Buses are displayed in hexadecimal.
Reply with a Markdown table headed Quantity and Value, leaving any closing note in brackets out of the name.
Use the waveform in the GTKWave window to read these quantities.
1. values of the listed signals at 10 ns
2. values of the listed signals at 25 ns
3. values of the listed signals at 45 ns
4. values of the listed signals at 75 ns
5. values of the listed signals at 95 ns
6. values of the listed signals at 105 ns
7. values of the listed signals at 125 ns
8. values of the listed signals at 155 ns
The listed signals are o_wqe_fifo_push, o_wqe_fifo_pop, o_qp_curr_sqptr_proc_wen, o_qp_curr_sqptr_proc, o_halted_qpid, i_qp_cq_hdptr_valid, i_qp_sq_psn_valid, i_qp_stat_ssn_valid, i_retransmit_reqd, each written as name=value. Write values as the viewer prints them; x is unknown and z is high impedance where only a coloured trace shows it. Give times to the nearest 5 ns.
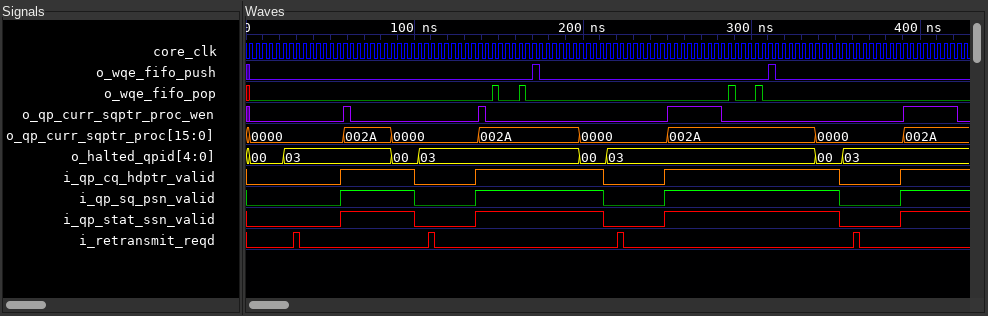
| Quantity | Value |
|---|---|
| values of the listed signals at 10 ns | o_wqe_fifo_push=0, o_wqe_fifo_pop=0, o_qp_curr_sqptr_proc_wen=0, o_qp_curr_sqptr_proc=0000, o_halted_qpid=00, i_qp_cq_hdptr_valid=0, i_qp_sq_psn_valid=0, i_qp_stat_ssn_valid=0, i_retransmit_reqd=0 |
| values of the listed signals at 25 ns | o_wqe_fifo_push=0, o_wqe_fifo_pop=0, o_qp_curr_sqptr_proc_wen=0, o_qp_curr_sqptr_proc=0000, o_halted_qpid=03, i_qp_cq_hdptr_valid=0, i_qp_sq_psn_valid=0, i_qp_stat_ssn_valid=0, i_retransmit_reqd=0 |
| values of the listed signals at 45 ns | o_wqe_fifo_push=0, o_wqe_fifo_pop=0, o_qp_curr_sqptr_proc_wen=0, o_qp_curr_sqptr_proc=0000, o_halted_qpid=03, i_qp_cq_hdptr_valid=0, i_qp_sq_psn_valid=0, i_qp_stat_ssn_valid=0, i_retransmit_reqd=0 |
| values of the listed signals at 75 ns | o_wqe_fifo_push=0, o_wqe_fifo_pop=0, o_qp_curr_sqptr_proc_wen=0, o_qp_curr_sqptr_proc=002A, o_halted_qpid=03, i_qp_cq_hdptr_valid=1, i_qp_sq_psn_valid=1, i_qp_stat_ssn_valid=1, i_retransmit_reqd=0 |
| values of the listed signals at 95 ns | o_wqe_fifo_push=0, o_wqe_fifo_pop=0, o_qp_curr_sqptr_proc_wen=0, o_qp_curr_sqptr_proc=0000, o_halted_qpid=00, i_qp_cq_hdptr_valid=1, i_qp_sq_psn_valid=1, i_qp_stat_ssn_valid=1, i_retransmit_reqd=0 |
| values of the listed signals at 105 ns | o_wqe_fifo_push=0, o_wqe_fifo_pop=0, o_qp_curr_sqptr_proc_wen=0, o_qp_curr_sqptr_proc=0000, o_halted_qpid=03, i_qp_cq_hdptr_valid=0, i_qp_sq_psn_valid=0, i_qp_stat_ssn_valid=0, i_retransmit_reqd=0 |
| values of the listed signals at 125 ns | o_wqe_fifo_push=0, o_wqe_fifo_pop=0, o_qp_curr_sqptr_proc_wen=0, o_qp_curr_sqptr_proc=0000, o_halted_qpid=03, i_qp_cq_hdptr_valid=0, i_qp_sq_psn_valid=0, i_qp_stat_ssn_valid=0, i_retransmit_reqd=0 |
| values of the listed signals at 155 ns | o_wqe_fifo_push=0, o_wqe_fifo_pop=0, o_qp_curr_sqptr_proc_wen=0, o_qp_curr_sqptr_proc=002A, o_halted_qpid=03, i_qp_cq_hdptr_valid=1, i_qp_sq_psn_valid=1, i_qp_stat_ssn_valid=1, i_retransmit_reqd=0 |
